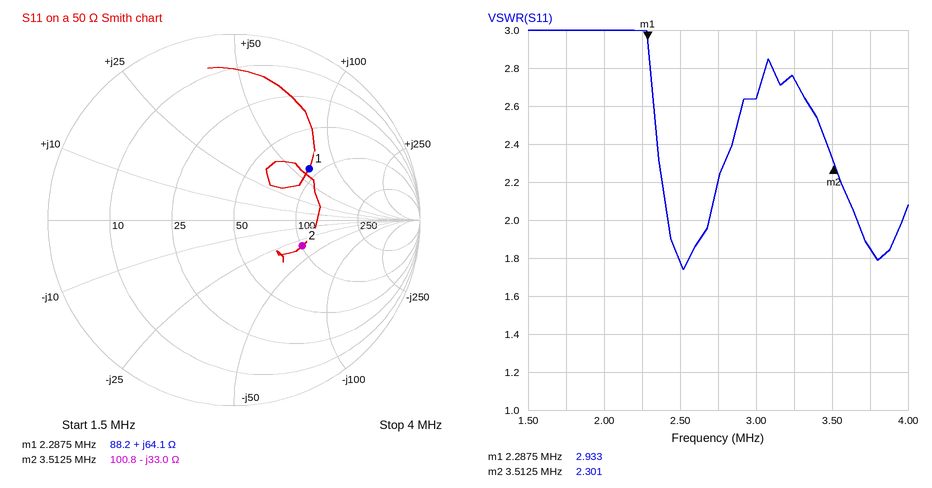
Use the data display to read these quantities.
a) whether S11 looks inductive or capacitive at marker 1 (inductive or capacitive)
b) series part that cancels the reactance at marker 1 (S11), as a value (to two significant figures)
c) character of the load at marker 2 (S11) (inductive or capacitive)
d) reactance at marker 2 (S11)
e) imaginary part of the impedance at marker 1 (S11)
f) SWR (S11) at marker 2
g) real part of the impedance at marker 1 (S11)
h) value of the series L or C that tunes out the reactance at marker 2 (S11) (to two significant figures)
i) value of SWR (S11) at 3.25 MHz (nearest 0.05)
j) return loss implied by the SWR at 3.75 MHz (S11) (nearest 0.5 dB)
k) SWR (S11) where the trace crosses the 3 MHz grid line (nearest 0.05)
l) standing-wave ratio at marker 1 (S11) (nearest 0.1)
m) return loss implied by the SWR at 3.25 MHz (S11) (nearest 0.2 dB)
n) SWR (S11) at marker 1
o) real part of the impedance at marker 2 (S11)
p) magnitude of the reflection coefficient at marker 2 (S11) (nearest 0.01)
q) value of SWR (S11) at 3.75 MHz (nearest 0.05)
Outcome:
inductive
1.1 nF
capacitive
-33.0 Ω
+64.1 Ω
2.301
88.2 Ω
1.5 µH
2.75
10.5 dB
2.65
2.9
6.6 dB
2.933
100.8 Ω
0.39
1.85
